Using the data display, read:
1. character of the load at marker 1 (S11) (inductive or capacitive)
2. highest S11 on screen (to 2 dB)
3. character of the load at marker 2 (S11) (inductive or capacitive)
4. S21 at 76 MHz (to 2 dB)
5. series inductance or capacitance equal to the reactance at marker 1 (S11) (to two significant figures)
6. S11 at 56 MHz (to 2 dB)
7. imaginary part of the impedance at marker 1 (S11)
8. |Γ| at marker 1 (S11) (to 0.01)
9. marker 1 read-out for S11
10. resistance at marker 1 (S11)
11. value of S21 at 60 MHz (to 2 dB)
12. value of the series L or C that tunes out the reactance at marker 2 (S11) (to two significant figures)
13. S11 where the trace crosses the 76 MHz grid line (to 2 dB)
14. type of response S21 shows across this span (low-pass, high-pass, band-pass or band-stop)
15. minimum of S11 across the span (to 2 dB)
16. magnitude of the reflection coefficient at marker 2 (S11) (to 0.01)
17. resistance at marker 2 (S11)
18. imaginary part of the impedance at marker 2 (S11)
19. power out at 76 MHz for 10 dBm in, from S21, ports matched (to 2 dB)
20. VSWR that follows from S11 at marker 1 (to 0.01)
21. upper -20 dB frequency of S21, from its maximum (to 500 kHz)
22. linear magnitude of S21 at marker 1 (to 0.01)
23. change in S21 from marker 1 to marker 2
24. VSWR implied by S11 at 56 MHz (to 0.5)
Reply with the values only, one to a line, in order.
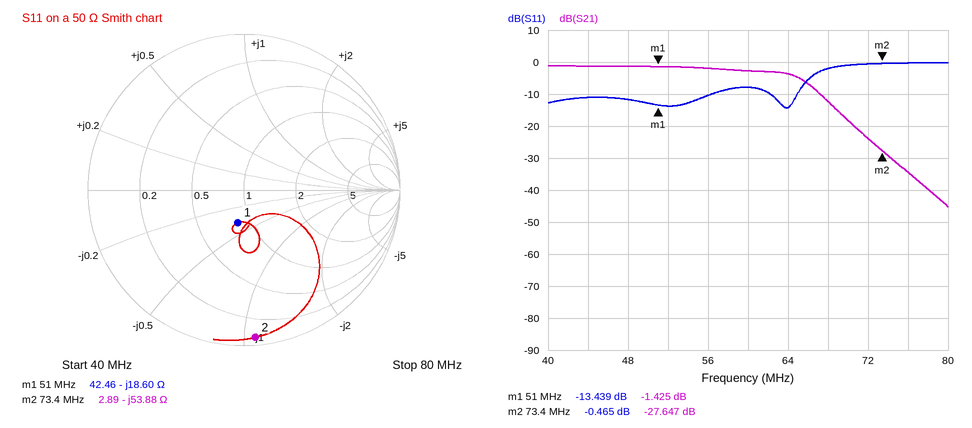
capacitive
0 dB
capacitive
-34 dB
170 pF
-10 dB
-18.60 Ω
0.21
-13.439 dB
42.46 Ω
-2 dB
120 nH
0 dB
low-pass
-14 dB
0.95
2.89 Ω
-53.88 Ω
-24 dBm
1.54
71.0 MHz
0.85
-26.222 dB
2.0
